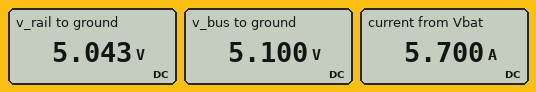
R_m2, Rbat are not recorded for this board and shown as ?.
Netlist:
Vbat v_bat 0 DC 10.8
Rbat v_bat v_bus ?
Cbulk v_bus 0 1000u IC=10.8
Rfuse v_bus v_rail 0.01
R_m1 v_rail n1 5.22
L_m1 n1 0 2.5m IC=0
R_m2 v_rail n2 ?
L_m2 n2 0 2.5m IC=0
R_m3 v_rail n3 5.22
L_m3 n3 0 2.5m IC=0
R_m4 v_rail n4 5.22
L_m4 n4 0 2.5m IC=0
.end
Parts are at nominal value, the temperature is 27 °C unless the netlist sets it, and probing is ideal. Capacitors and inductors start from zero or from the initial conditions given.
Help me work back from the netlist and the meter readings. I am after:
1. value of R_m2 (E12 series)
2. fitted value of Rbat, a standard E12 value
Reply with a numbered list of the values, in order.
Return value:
1. 1.8 Ω
2. 1 Ω
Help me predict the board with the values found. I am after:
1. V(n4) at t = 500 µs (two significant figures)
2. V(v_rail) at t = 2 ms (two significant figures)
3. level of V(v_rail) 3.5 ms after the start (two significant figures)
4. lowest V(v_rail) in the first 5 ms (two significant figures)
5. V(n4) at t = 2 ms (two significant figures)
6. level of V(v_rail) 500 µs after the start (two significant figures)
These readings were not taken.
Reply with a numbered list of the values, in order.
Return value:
1. 2.8 V
2. 5.2 V
3. 5.0 V
4. 4.9 V
5. -730 mV
6. 9.4 V
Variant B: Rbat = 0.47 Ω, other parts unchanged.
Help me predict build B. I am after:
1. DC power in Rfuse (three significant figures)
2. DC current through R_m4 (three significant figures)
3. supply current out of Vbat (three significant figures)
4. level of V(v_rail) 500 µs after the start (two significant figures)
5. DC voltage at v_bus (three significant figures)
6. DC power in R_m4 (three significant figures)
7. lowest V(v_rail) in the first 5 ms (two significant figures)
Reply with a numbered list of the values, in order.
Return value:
1. 626 mW
2. 1.34 A
3. 7.91 A
4. 9.6 V
5. 7.08 V
6. 9.39 W
7. 7.0 V
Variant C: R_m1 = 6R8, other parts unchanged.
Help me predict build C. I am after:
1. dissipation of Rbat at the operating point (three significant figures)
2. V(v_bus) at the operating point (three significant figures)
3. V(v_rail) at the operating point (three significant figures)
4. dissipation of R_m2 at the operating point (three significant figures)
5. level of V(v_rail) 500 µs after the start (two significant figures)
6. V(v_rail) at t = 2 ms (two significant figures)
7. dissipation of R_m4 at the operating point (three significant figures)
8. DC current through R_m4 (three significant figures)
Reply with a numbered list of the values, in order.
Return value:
1. 31.3 W
2. 5.21 V
3. 5.15 V
4. 14.7 W
5. 9.4 V
6. 5.4 V
7. 5.08 W
8. 987 mA
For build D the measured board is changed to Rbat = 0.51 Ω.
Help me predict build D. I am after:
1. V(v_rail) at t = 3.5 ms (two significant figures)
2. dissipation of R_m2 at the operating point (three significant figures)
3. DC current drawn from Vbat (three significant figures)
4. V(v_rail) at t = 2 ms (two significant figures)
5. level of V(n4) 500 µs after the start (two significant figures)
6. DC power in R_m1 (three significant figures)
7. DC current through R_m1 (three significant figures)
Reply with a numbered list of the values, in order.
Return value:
1. 6.8 V
2. 25.7 W
3. 7.69 A
4. 7.0 V
5. 3.0 V
6. 8.86 W
7. 1.30 A
